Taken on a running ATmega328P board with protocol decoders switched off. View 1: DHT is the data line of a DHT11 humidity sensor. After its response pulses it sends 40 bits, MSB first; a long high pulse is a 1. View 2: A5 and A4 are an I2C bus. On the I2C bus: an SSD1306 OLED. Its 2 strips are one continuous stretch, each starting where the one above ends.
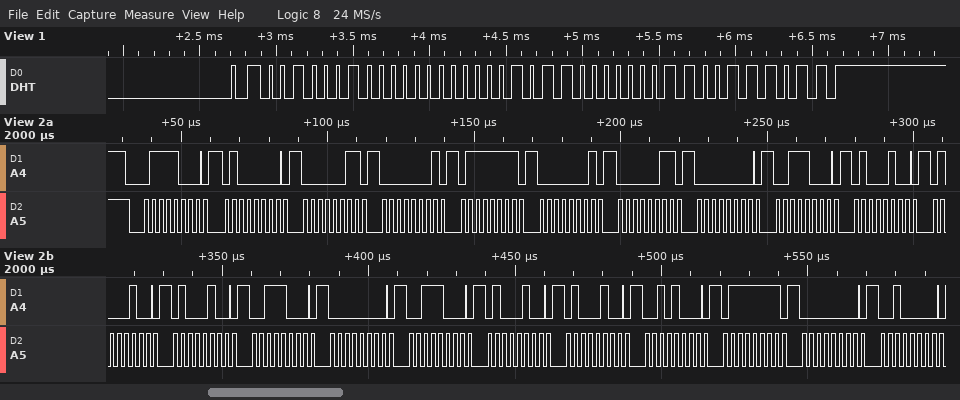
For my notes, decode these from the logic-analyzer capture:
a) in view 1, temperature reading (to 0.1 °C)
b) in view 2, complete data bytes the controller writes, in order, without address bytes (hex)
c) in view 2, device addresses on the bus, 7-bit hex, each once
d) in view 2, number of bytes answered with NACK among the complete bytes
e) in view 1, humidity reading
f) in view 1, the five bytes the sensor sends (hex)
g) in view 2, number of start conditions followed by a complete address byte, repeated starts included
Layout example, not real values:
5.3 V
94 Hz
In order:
22.3 °C
40 03 01 7F 01 03 00 38 44 44 44 38 00 38 44 44 28 7F 00 20
0x3C
0
34 %
22 00 16 03 3B
1
